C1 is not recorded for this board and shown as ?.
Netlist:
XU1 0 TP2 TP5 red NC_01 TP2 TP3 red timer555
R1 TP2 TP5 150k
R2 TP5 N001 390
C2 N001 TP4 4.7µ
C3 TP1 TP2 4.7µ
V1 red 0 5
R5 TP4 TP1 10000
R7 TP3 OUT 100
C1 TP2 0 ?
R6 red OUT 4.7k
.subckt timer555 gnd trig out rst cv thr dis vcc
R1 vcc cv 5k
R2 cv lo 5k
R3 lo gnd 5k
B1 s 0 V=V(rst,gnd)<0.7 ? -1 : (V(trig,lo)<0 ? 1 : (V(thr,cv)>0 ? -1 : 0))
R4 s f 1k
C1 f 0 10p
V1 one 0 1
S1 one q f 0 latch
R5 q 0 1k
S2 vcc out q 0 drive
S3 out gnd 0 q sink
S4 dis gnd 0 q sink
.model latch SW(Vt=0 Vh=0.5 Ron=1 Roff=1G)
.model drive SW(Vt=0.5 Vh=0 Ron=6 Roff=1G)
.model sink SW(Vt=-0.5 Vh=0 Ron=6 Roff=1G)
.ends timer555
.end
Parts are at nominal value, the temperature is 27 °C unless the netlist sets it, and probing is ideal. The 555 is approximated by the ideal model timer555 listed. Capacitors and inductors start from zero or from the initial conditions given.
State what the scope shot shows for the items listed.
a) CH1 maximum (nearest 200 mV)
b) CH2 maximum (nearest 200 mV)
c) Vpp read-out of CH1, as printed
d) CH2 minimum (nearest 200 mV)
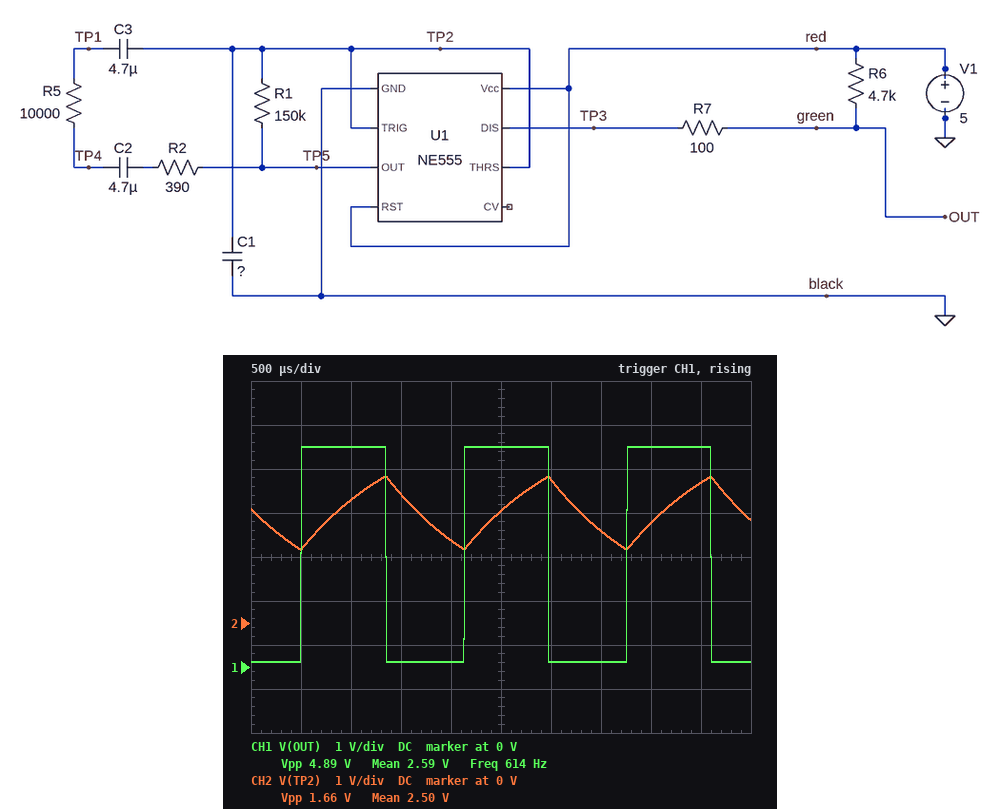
5.0 V
3.4 V
4.89 V
1.6 V
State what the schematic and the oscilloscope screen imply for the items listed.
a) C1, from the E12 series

120 nF
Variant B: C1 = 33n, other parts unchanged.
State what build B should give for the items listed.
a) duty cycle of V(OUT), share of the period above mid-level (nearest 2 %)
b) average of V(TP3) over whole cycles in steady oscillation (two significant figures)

50 %
2.5 V
